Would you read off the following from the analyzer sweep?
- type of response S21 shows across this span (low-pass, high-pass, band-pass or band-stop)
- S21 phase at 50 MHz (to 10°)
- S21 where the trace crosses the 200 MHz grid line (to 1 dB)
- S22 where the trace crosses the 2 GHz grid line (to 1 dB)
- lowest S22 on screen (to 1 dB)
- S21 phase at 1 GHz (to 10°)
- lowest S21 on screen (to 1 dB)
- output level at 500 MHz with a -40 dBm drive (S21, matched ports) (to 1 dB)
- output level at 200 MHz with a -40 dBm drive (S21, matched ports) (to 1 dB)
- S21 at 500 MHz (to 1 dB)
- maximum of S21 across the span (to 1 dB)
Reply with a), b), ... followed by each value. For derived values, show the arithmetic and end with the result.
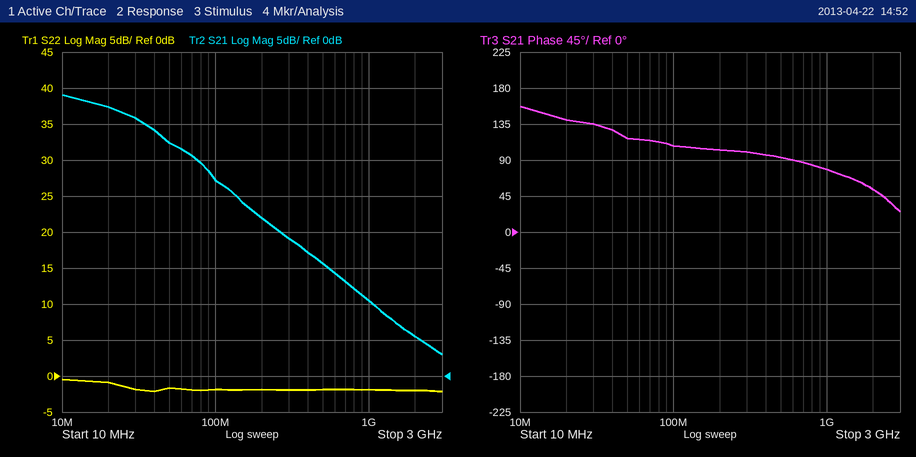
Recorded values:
a) low-pass
b) 120°
c) 22 dB
d) -2 dB
e) -2 dB
f) 80°
g) 3 dB
h) -40 dBm + (16 dB) = -24 dBm
i) -40 dBm + (22 dB) = -18 dBm
j) 16 dB
k) 39 dB
